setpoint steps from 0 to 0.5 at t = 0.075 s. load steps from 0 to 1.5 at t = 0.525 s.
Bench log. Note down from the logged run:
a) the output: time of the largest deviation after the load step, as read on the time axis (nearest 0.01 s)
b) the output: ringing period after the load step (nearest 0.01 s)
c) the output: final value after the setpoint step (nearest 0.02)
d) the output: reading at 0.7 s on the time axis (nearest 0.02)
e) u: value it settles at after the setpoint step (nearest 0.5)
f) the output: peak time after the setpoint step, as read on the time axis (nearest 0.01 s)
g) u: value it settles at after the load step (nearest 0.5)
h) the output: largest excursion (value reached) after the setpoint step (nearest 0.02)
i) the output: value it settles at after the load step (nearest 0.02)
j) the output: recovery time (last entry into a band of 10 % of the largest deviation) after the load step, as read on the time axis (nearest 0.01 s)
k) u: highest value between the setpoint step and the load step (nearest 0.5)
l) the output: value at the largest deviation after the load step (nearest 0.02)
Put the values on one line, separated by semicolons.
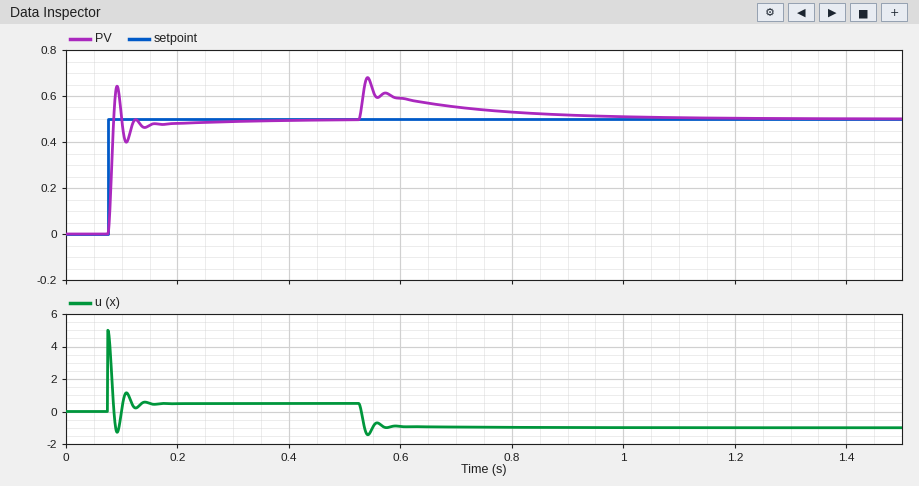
0.54 s; 0.03 s; 0.50; 0.56; 0.5; 0.09 s; -1.0; 0.64; 0.50; 0.89 s; 5.0; 0.68
